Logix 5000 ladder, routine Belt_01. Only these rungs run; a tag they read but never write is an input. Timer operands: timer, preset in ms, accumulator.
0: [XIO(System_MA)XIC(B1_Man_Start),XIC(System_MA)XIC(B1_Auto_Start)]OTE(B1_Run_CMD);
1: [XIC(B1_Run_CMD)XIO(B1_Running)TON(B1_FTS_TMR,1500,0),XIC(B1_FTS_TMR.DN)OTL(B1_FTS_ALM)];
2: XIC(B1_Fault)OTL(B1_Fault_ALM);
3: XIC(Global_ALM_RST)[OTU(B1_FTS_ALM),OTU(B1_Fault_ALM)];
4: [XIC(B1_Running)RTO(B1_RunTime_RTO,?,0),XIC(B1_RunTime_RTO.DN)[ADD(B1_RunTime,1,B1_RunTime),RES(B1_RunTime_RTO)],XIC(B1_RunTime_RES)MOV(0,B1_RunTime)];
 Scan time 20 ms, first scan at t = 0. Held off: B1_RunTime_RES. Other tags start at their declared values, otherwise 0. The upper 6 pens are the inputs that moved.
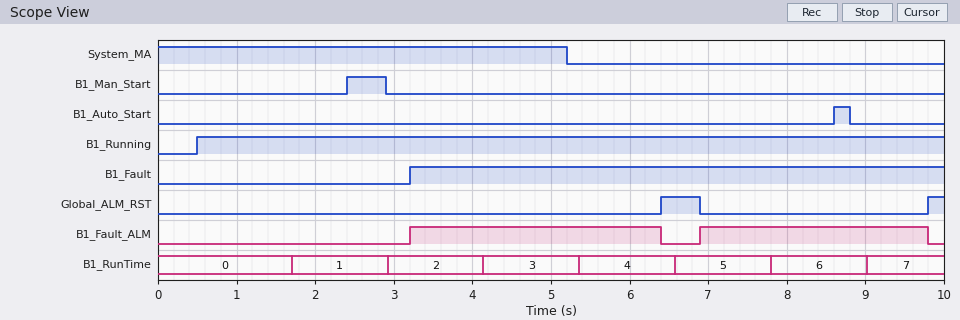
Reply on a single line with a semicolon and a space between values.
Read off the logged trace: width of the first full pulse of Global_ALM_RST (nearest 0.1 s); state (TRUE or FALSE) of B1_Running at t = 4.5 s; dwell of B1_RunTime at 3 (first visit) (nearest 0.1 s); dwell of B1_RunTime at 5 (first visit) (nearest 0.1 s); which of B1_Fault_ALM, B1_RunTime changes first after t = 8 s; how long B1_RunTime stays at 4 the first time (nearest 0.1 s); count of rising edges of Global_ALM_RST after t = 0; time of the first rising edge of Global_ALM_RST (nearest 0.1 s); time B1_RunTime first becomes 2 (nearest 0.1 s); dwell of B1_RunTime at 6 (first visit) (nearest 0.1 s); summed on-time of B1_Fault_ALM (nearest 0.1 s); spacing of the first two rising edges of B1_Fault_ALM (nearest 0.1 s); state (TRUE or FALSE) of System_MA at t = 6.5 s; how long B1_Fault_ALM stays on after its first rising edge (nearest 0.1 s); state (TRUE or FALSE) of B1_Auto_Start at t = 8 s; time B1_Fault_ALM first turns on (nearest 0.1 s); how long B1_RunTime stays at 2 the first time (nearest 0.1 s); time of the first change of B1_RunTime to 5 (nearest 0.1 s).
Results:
0.5 s; TRUE; 1.2 s; 1.2 s; B1_RunTime; 1.2 s; 2; 6.4 s; 2.9 s; 1.2 s; 6.1 s; 3.7 s; FALSE; 3.2 s; FALSE; 3.2 s; 1.2 s; 6.6 s
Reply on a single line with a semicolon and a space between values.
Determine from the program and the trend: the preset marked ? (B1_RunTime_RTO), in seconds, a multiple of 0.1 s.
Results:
1.2 s
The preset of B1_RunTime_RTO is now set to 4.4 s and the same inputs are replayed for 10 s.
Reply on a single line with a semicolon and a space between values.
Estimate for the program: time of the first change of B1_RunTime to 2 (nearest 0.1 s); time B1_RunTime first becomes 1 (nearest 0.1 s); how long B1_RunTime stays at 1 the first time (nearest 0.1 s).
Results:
9.3 s; 4.9 s; 4.4 s
